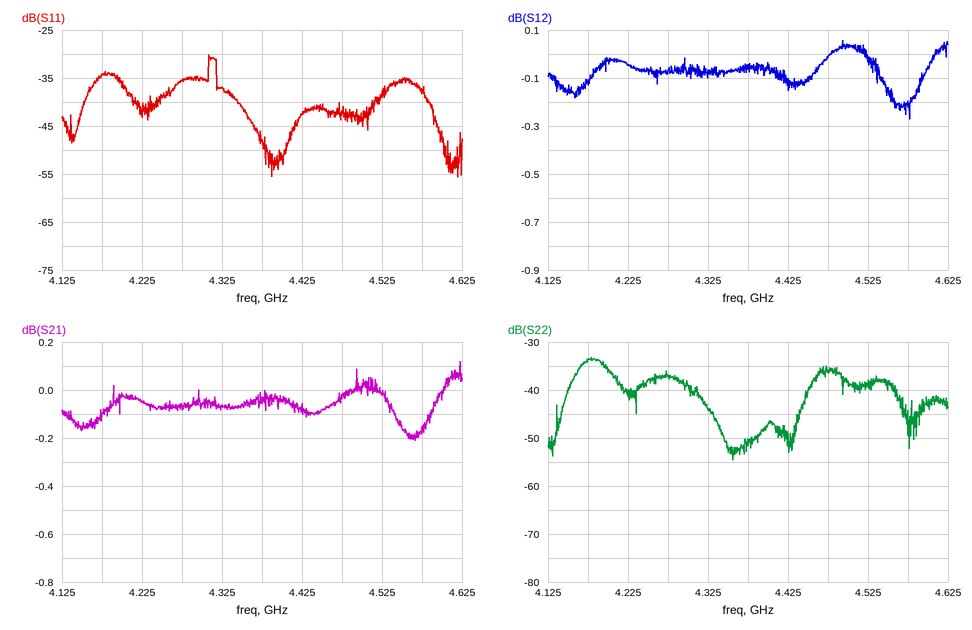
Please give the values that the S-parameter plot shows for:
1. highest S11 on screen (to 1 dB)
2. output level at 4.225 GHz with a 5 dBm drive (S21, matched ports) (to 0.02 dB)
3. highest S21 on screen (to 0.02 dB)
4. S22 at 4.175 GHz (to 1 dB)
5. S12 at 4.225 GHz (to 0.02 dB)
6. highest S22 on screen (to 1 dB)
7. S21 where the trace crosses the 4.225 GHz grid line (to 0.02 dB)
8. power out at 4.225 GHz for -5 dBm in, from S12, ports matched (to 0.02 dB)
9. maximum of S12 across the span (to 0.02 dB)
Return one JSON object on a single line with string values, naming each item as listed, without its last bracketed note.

{"highest S11 on screen": "-30 dB", "output level at 4.225 GHz with a 5 dBm drive (S21, matched ports)": "4.96 dBm", "highest S21 on screen": "0.12 dB", "S22 at 4.175 GHz": "-34 dB", "S12 at 4.225 GHz": "-0.04 dB", "highest S22 on screen": "-33 dB", "S21 where the trace crosses the 4.225 GHz grid line": "-0.04 dB", "power out at 4.225 GHz for -5 dBm in, from S12, ports matched": "-5.04 dBm", "maximum of S12 across the span": "0.06 dB"}
